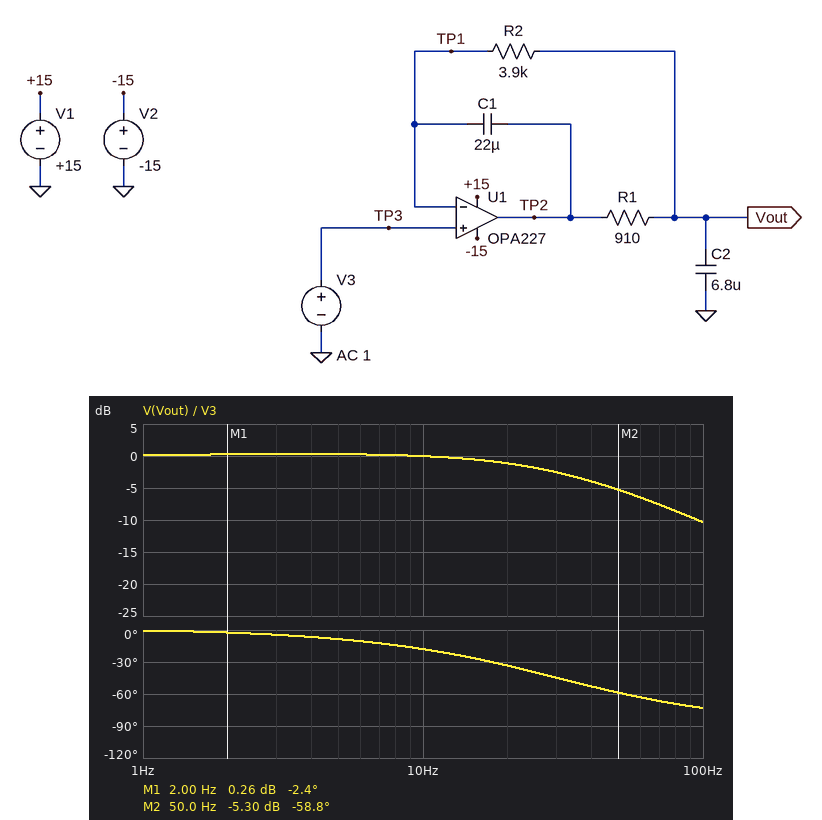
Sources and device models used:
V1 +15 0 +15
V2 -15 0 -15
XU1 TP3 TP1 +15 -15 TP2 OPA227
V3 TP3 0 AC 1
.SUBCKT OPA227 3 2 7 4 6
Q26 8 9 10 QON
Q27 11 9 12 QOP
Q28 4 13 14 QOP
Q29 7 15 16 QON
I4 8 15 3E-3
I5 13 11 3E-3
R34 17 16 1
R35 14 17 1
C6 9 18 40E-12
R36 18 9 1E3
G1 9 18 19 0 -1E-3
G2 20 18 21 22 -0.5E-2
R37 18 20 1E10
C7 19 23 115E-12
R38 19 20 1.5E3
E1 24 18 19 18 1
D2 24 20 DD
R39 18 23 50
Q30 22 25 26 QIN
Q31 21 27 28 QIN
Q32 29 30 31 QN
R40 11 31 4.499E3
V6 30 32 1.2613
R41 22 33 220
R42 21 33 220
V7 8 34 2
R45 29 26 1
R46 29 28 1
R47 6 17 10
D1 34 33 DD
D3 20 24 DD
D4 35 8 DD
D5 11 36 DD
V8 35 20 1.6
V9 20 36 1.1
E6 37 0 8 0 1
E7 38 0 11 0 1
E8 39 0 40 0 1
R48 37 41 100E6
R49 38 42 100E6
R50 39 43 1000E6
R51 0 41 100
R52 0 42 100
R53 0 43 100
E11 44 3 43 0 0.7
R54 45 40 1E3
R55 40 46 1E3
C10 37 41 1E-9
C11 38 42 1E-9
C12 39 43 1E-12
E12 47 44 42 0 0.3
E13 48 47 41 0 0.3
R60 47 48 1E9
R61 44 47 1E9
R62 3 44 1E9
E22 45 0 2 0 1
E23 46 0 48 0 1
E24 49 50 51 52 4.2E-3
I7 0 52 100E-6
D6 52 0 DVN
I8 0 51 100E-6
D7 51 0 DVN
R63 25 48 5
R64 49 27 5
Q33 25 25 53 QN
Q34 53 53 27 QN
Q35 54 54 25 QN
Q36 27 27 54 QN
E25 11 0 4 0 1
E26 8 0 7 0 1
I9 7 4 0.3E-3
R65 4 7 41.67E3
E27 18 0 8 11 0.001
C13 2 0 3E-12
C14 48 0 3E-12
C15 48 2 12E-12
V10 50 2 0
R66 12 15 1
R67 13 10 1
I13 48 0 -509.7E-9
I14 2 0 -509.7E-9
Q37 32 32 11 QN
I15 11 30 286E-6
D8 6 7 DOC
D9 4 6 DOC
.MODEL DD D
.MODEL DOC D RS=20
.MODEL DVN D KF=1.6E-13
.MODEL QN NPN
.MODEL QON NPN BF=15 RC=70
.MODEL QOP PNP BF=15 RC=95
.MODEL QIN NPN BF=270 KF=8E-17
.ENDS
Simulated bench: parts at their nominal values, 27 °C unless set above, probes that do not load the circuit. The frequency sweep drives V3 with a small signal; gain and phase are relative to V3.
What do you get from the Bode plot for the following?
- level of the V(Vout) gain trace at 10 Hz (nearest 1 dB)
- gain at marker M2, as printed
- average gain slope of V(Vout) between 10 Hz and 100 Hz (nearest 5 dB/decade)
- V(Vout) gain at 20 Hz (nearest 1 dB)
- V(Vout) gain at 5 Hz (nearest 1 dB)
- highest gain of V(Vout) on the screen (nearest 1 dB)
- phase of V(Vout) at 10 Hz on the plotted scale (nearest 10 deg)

0 dB
-5.30 dB
-10 dB/decade
-1 dB
0 dB
0 dB
-20 deg
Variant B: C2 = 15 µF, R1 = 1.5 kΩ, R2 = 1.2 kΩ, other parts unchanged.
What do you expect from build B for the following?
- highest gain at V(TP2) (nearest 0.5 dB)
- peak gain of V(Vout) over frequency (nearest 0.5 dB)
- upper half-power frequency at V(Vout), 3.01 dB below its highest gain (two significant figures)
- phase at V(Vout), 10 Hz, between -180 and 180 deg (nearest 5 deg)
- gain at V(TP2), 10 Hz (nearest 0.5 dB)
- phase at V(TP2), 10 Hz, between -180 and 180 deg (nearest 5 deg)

3.0 dB
1.0 dB
16 Hz
-35 deg
2.5 dB
-5 deg
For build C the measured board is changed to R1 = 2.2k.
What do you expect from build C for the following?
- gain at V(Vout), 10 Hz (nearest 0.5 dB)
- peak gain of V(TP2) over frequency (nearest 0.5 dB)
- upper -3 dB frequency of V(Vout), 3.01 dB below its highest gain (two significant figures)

-1.0 dB
1.0 dB
16 Hz
